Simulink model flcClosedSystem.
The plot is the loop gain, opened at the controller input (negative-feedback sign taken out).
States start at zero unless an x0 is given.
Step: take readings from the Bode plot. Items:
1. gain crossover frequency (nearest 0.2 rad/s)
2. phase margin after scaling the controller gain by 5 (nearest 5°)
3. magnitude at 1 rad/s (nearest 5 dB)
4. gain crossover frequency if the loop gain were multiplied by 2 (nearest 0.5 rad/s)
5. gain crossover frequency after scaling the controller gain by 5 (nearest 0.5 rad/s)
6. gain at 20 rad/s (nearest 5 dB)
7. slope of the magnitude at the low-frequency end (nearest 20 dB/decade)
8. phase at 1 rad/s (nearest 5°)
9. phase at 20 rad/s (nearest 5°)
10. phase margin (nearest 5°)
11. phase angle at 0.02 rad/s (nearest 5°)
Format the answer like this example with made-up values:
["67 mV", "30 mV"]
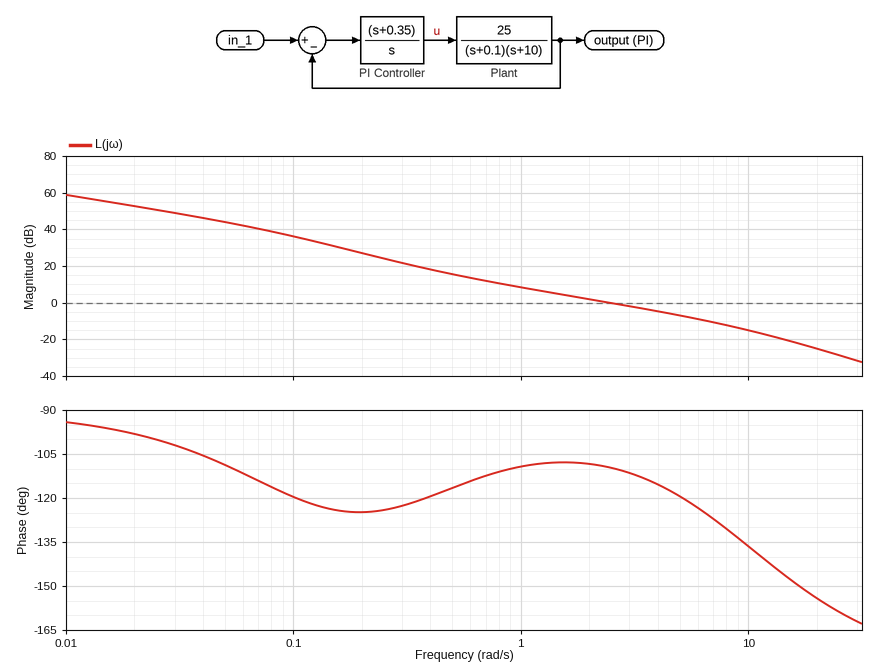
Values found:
["2.4 rad/s", "45°", "10 dB", "4.5 rad/s", "9.0 rad/s", "-25 dB", "-20 dB/decade", "-110°", "-155°", "70°", "-100°"]
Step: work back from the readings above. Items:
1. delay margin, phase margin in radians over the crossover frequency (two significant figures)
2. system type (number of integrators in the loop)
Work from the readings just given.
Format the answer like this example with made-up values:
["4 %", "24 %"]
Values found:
["0.51 s", "1"]
